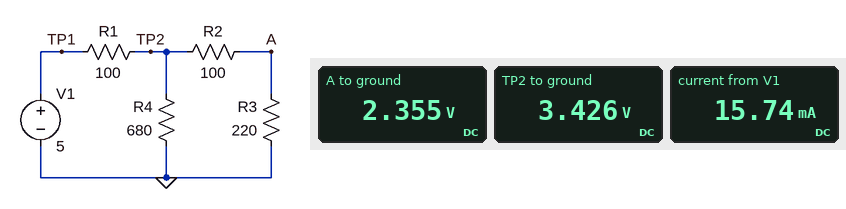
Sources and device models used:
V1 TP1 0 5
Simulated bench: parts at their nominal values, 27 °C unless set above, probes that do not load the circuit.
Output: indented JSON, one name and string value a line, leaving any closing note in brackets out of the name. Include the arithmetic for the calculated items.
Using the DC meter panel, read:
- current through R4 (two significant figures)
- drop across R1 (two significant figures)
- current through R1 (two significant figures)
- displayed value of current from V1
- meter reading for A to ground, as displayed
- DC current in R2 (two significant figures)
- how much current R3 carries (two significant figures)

{
  "current through R4": "(3.426 V) / 680 Ω = 5.0 mA",
  "drop across R1": "5 V - 3.426 V = 1.6 V",
  "current through R1": "(5 V - 3.426 V) / 100 Ω = 16 mA",
  "displayed value of current from V1": "15.74 mA",
  "meter reading for A to ground, as displayed": "2.355 V",
  "DC current in R2": "(3.426 V - 2.355 V) / 100 Ω = 11 mA",
  "how much current R3 carries": "(2.355 V) / 220 Ω = 11 mA"
}
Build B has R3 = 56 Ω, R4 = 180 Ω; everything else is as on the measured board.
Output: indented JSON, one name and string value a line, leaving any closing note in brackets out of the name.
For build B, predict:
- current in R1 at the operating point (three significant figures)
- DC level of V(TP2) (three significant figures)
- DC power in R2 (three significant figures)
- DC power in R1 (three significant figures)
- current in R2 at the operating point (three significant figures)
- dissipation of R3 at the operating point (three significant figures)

{
  "current in R1 at the operating point": "27.2 mA",
  "DC level of V(TP2)": "2.28 V",
  "DC power in R2": "21.3 mW",
  "DC power in R1": "74.2 mW",
  "current in R2 at the operating point": "14.6 mA",
  "dissipation of R3 at the operating point": "11.9 mW"
}
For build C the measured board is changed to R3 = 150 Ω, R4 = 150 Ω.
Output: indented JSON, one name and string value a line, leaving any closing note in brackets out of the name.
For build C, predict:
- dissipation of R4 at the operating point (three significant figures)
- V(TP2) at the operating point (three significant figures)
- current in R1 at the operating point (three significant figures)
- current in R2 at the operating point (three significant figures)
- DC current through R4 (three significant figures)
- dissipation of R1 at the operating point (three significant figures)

{
  "dissipation of R4 at the operating point": "39.0 mW",
  "V(TP2) at the operating point": "2.42 V",
  "current in R1 at the operating point": "25.8 mA",
  "current in R2 at the operating point": "9.68 mA",
  "DC current through R4": "16.1 mA",
  "dissipation of R1 at the operating point": "66.6 mW"
}
